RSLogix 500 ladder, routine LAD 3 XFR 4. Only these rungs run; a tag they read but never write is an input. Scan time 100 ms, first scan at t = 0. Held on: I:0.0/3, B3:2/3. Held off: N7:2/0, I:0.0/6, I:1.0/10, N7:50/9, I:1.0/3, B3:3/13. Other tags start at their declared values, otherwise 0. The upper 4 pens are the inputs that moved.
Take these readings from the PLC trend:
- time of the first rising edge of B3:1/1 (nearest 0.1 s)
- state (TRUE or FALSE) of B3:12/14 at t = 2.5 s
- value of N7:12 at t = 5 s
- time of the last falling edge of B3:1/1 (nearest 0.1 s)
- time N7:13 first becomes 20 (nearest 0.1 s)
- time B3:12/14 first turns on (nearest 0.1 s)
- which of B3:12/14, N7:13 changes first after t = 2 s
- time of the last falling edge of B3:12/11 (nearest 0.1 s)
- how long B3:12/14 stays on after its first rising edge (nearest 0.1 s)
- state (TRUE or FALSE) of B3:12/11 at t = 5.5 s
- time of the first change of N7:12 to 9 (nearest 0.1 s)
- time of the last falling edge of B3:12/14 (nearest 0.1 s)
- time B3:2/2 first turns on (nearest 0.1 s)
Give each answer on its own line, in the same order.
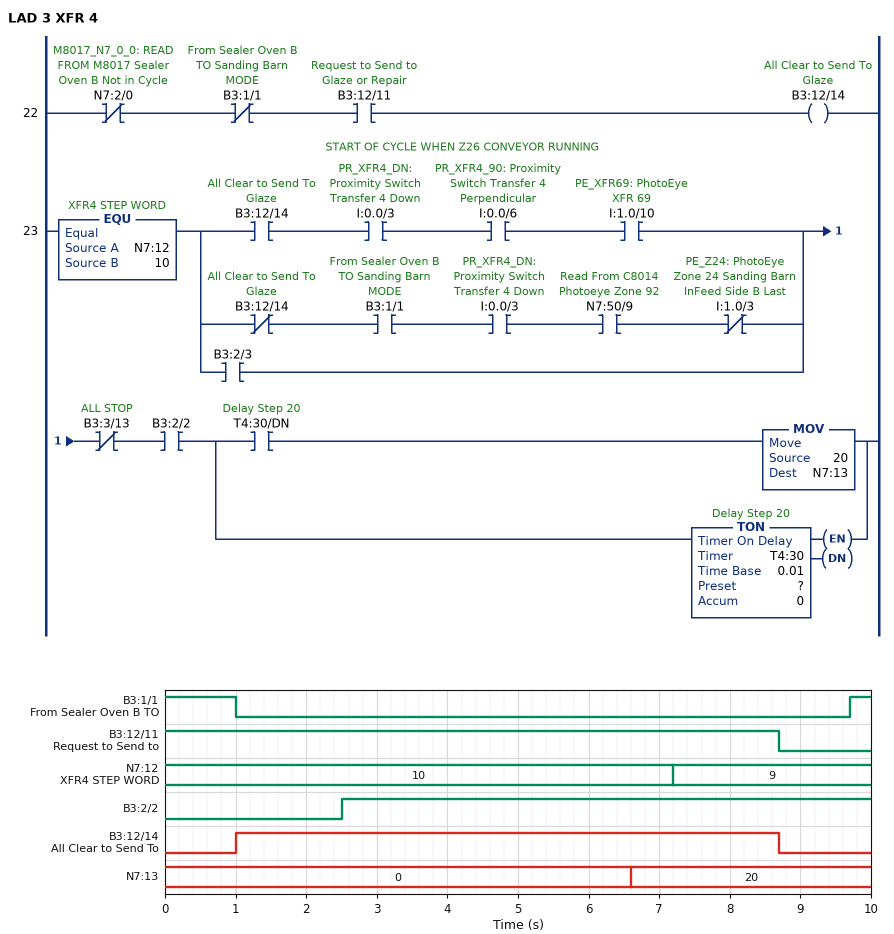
9.7 s
TRUE
10
1.0 s
6.6 s
1.0 s
N7:13
8.7 s
7.7 s
TRUE
7.2 s
8.7 s
2.5 s
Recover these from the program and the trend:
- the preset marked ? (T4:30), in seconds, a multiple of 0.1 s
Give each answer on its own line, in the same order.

4.0 s
